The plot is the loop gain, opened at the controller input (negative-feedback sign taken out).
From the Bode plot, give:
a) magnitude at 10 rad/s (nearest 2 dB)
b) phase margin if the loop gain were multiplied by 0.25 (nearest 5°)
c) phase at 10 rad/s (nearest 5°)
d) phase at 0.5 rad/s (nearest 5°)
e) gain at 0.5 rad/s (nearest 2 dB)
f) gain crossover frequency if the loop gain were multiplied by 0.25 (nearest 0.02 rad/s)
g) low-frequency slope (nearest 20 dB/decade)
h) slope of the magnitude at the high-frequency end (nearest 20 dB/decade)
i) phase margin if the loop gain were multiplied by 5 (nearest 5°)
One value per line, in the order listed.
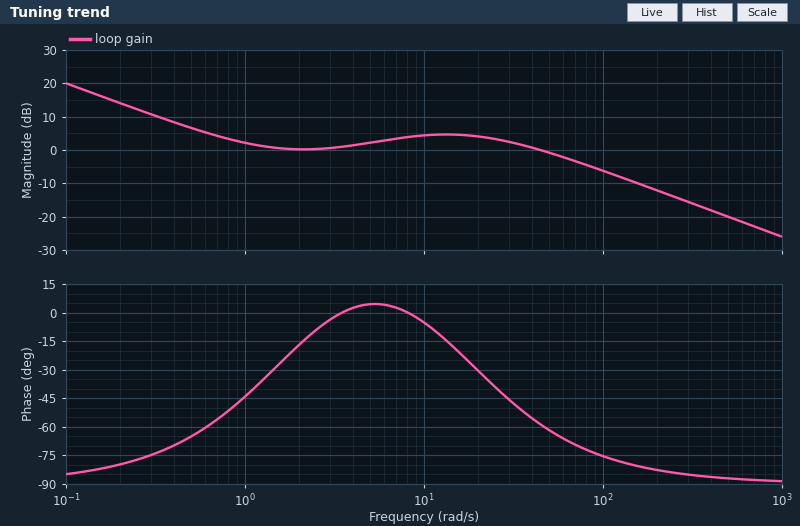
4 dB
105°
-5°
-65°
6 dB
0.26 rad/s
-20 dB/decade
-20 dB/decade
95°
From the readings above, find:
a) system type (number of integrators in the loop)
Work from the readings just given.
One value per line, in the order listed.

1
